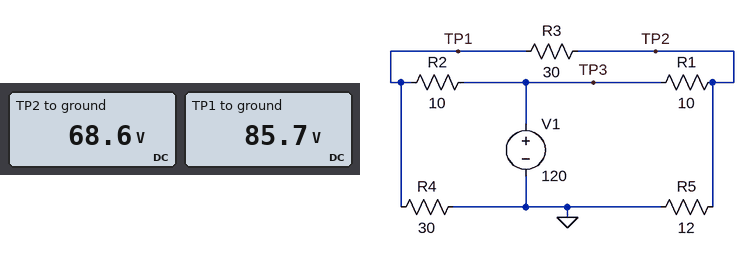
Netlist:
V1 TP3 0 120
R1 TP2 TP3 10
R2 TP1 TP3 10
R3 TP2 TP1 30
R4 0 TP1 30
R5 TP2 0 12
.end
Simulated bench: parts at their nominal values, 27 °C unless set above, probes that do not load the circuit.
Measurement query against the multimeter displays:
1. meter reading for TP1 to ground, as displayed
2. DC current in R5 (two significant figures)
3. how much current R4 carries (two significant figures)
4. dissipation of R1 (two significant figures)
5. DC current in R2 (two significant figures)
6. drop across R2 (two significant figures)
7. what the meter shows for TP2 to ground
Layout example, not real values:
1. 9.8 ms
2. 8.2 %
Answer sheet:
1. 85.7 V
2. 5.7 A
3. 2.9 A
4. 260 W
5. 3.4 A
6. 34 V
7. 68.6 V
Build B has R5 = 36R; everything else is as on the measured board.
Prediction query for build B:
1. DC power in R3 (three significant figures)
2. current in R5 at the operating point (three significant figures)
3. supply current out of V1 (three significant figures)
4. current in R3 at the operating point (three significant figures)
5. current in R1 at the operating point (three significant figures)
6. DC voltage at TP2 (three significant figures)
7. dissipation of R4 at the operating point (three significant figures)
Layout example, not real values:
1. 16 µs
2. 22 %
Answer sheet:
1. 224 mW
2. 2.59 A
3. 5.61 A
4. 86.3 mA
5. 2.68 A
6. 93.2 V
7. 274 W
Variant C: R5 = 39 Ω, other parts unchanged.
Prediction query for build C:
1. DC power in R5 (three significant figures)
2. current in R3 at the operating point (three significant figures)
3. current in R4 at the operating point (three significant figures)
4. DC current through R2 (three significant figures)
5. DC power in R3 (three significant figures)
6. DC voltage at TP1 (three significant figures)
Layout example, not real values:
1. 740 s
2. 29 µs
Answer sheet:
1. 229 W
2. 121 mA
3. 3.03 A
4. 2.91 A
5. 441 mW
6. 90.9 V
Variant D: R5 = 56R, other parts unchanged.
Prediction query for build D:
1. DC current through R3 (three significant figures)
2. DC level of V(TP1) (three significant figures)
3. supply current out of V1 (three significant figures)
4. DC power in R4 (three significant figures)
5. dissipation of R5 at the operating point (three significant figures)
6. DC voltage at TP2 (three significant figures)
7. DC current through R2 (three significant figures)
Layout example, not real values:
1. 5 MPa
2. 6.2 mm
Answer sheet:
1. 257 mA
2. 91.9 V
3. 4.84 A
4. 282 W
5. 177 W
6. 99.6 V
7. 2.81 A
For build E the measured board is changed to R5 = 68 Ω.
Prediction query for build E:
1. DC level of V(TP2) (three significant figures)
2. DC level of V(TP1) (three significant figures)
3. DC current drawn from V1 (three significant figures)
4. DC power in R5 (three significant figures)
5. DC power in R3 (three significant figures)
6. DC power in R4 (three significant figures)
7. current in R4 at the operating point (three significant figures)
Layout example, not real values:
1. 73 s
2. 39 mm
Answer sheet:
1. 102 V
2. 92.4 V
3. 4.58 A
4. 153 W
5. 3.00 W
6. 284 W
7. 3.08 A
